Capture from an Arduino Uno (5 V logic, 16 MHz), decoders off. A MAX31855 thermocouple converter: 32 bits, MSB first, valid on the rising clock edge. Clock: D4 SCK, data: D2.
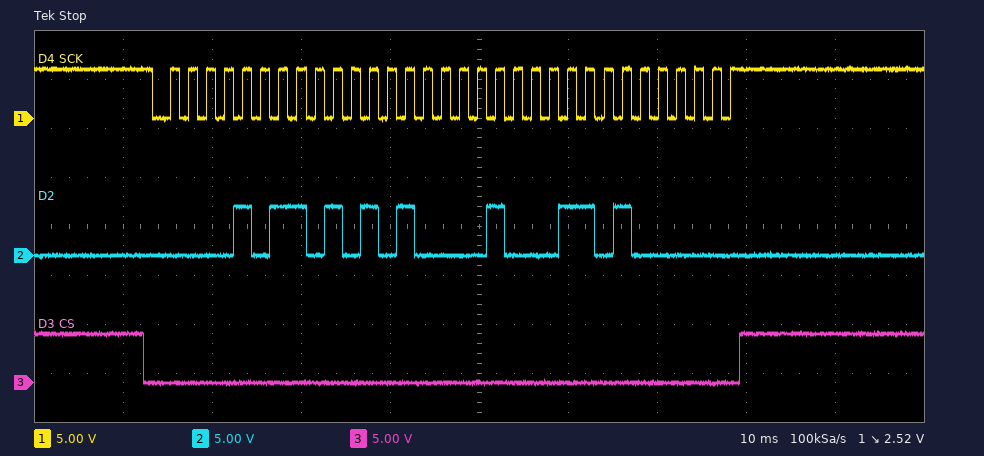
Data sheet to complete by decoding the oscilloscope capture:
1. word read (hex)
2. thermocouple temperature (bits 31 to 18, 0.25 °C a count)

0x0B542340
181.25 °C
